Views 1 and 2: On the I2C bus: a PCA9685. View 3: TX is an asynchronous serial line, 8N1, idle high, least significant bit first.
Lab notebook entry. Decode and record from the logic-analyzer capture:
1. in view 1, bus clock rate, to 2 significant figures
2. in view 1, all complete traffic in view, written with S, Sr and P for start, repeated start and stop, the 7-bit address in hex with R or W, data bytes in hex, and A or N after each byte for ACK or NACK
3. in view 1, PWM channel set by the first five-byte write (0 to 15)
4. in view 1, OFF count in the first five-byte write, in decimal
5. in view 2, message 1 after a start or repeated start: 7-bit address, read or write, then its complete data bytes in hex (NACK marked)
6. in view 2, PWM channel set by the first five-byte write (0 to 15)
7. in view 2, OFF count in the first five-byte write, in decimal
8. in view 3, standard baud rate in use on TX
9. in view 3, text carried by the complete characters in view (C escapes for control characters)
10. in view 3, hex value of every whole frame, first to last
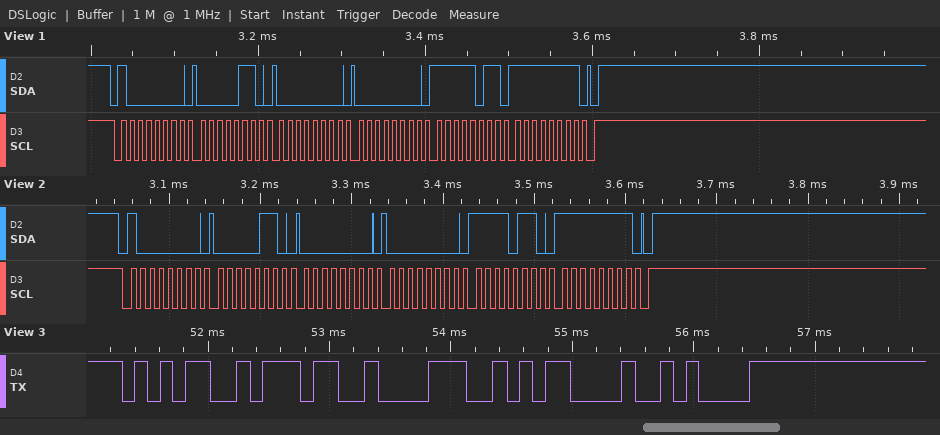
100 kHz
S 40W A 06 A 00 A 00 A FB A FF A P
0
65531
0x40 write: 06 00 00 F6 FF
0
65526
9600 baud
"578\r\n"
35 37 38 0D 0A
